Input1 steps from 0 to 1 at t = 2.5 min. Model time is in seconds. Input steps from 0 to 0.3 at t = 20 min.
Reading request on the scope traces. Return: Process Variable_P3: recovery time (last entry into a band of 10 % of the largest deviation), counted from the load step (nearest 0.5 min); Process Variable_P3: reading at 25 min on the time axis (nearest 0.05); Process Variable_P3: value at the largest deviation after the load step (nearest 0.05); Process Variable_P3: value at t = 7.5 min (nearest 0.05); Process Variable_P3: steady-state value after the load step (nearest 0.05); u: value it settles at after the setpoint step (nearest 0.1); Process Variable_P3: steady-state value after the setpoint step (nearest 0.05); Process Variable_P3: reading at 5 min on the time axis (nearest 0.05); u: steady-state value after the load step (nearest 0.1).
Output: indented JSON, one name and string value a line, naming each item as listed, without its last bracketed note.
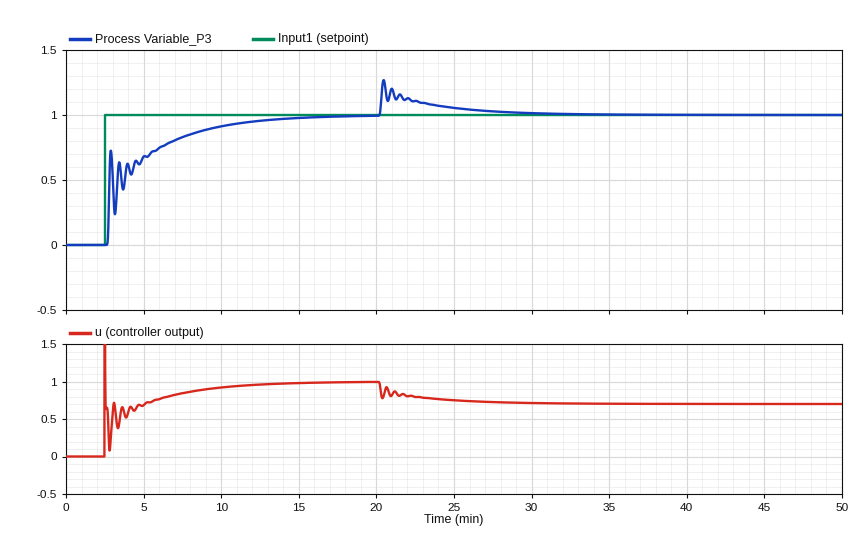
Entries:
{
  "Process Variable_P3: recovery time (last entry into a band of 10 % of the largest deviation), counted from the load step": "7.5 min",
  "Process Variable_P3: reading at 25 min on the time axis": "1.05",
  "Process Variable_P3: value at the largest deviation after the load step": "1.25",
  "Process Variable_P3: value at t = 7.5 min": "0.85",
  "Process Variable_P3: steady-state value after the load step": "1.00",
  "u: value it settles at after the setpoint step": "1.0",
  "Process Variable_P3: steady-state value after the setpoint step": "1.00",
  "Process Variable_P3: reading at 5 min on the time axis": "0.70",
  "u: steady-state value after the load step": "0.7"
}
